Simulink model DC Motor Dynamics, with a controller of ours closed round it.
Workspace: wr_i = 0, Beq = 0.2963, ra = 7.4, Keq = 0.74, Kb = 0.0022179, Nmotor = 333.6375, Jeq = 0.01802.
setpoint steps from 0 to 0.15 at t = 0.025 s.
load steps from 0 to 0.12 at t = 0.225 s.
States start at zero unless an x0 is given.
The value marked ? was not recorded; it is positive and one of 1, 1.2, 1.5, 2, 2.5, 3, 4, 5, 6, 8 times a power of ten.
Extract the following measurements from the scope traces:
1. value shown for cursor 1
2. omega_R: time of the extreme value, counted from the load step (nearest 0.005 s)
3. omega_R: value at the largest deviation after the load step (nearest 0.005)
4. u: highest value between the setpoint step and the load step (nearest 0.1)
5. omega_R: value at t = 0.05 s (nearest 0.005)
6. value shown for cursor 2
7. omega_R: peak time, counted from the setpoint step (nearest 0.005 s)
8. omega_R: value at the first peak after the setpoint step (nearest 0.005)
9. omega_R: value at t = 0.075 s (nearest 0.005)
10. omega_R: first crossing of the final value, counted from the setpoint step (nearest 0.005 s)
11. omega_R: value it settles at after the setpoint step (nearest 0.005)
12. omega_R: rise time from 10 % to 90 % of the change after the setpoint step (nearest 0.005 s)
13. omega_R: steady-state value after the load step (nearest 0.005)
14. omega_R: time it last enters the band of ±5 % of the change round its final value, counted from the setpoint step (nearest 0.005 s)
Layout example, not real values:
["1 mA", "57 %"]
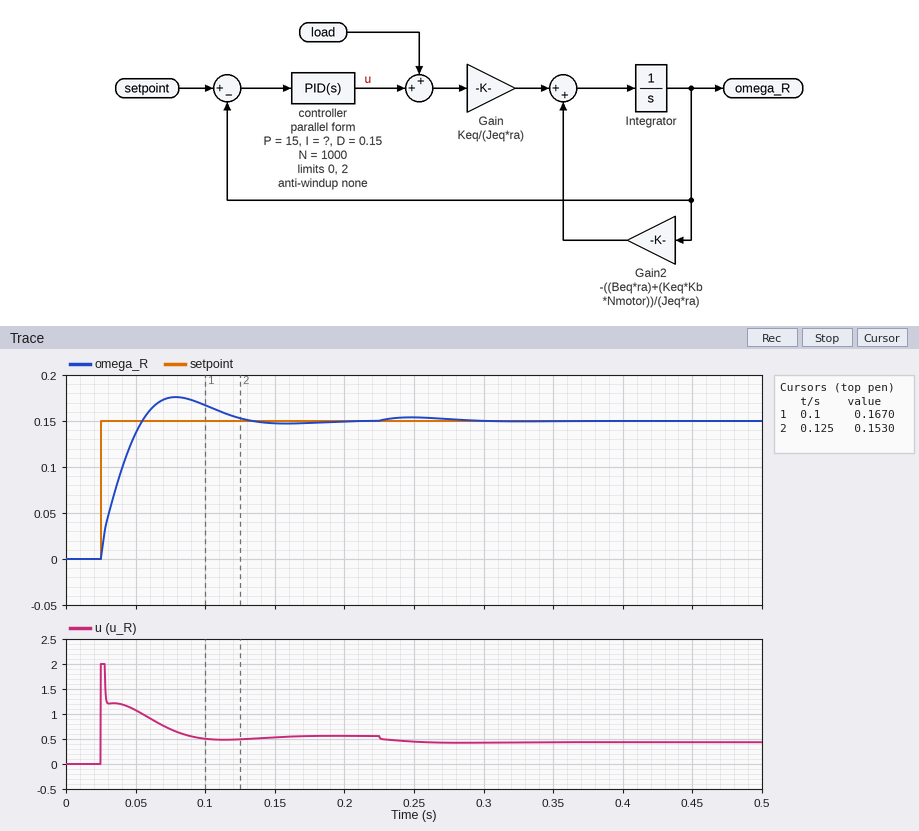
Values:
["0.1670", "0.025 s", "0.155", "2.0", "0.135", "0.1530", "0.055 s", "0.175", "0.175", "0.030 s", "0.150", "0.025 s", "0.150", "0.090 s"]
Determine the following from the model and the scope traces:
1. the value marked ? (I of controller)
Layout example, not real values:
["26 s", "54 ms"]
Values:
["800"]
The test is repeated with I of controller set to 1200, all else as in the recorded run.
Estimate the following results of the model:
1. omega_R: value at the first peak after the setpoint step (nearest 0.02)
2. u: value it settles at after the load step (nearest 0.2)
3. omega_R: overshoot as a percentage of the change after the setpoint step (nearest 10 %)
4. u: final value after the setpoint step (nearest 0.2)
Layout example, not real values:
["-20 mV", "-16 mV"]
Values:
["0.18", "0.4", "20 %", "0.6"]
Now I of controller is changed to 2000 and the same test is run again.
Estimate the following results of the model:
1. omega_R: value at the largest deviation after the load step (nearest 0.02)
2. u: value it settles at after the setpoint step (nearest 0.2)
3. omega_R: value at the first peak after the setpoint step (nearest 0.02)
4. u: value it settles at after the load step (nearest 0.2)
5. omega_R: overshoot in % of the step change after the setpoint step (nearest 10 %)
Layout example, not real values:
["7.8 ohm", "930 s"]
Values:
["0.16", "0.6", "0.20", "0.4", "30 %"]
